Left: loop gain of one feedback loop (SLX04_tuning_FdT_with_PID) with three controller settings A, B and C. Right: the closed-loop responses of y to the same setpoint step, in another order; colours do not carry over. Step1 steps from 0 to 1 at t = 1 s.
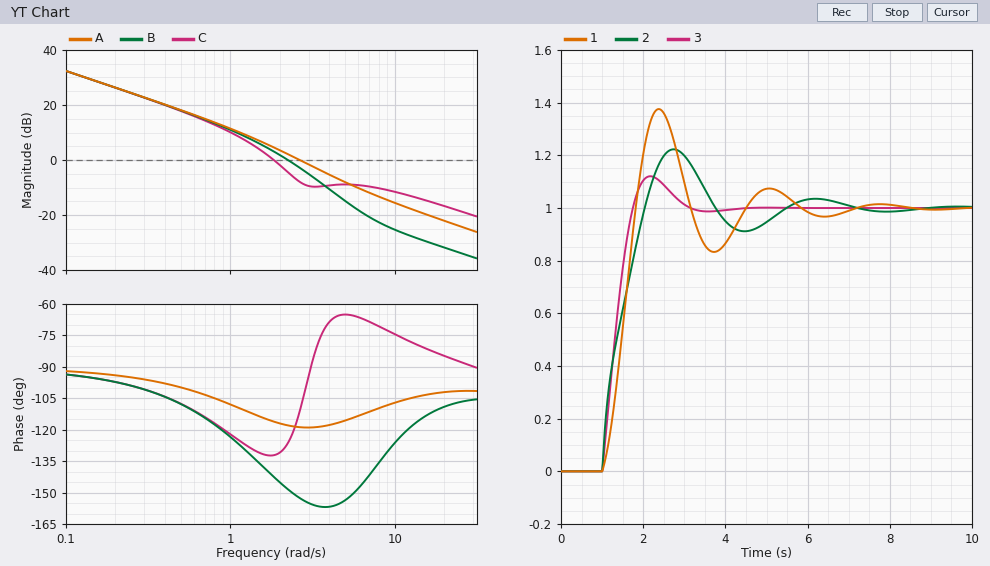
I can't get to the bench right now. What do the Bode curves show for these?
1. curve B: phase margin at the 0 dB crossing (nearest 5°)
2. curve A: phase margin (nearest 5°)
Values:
30°
60°
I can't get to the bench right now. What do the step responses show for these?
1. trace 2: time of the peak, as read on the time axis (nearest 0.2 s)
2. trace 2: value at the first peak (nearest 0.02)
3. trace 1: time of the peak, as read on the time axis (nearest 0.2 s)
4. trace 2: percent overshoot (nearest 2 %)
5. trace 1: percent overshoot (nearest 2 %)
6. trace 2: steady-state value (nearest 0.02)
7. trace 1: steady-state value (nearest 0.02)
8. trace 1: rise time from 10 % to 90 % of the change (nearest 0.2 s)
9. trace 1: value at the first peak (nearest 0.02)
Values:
2.8 s
1.22
2.4 s
22 %
38 %
1.00
1.00
0.6 s
1.38
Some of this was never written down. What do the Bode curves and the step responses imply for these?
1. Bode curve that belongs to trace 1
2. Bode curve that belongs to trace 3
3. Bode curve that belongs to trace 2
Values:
B
A
C
